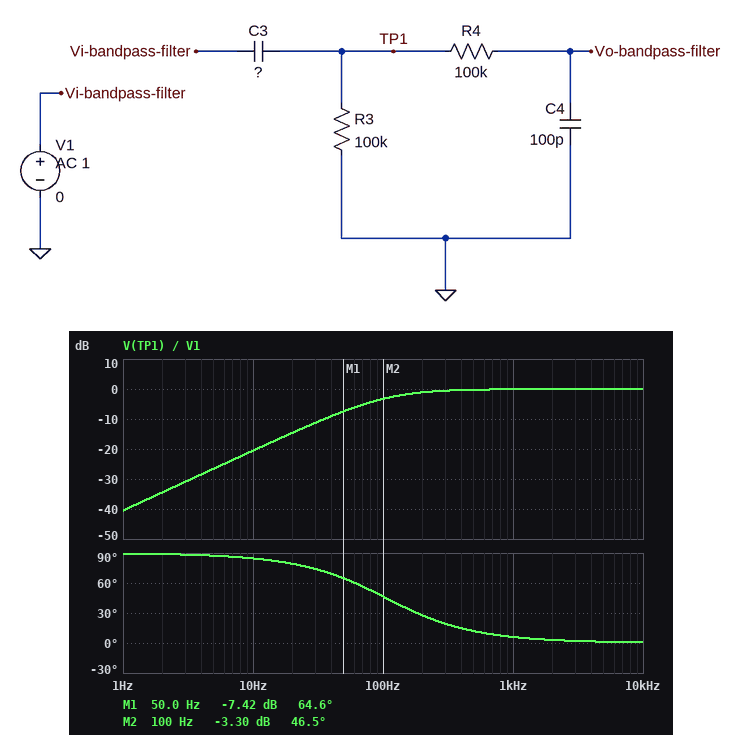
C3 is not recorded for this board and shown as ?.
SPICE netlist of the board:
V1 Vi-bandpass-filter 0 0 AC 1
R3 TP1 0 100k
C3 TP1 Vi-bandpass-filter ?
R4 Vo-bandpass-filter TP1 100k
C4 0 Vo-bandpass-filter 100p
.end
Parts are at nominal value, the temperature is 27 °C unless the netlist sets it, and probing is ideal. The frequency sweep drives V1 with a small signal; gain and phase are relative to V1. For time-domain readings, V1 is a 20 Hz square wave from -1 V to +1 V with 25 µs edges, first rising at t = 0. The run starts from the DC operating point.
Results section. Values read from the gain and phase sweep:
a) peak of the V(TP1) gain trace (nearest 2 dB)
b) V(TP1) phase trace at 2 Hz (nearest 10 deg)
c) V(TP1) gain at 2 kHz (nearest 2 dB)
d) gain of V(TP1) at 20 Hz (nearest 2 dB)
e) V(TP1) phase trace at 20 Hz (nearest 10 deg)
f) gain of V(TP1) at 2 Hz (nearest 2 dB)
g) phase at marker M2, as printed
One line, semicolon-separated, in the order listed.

0 dB; 90 deg; 0 dB; -14 dB; 80 deg; -34 dB; 46.5 deg
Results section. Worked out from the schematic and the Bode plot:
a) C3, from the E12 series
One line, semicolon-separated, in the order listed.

15 nF
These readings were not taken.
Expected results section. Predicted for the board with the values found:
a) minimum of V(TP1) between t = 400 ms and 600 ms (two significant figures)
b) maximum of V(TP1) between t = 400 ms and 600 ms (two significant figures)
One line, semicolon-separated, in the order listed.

-2.0 V; 2.0 V
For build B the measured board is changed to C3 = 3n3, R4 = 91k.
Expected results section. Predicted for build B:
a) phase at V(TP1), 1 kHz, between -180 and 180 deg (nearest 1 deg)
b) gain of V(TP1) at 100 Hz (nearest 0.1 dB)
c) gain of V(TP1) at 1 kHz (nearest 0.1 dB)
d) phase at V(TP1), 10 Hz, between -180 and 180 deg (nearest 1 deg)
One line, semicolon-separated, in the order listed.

25 deg; -13.9 dB; -1.1 dB; 89 deg
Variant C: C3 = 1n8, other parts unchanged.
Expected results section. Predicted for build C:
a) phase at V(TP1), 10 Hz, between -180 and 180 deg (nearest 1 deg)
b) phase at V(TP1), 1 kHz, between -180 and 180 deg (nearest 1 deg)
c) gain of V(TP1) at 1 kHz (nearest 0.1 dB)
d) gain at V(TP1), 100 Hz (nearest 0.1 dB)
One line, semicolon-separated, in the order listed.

89 deg; 40 deg; -2.8 dB; -19.0 dB
